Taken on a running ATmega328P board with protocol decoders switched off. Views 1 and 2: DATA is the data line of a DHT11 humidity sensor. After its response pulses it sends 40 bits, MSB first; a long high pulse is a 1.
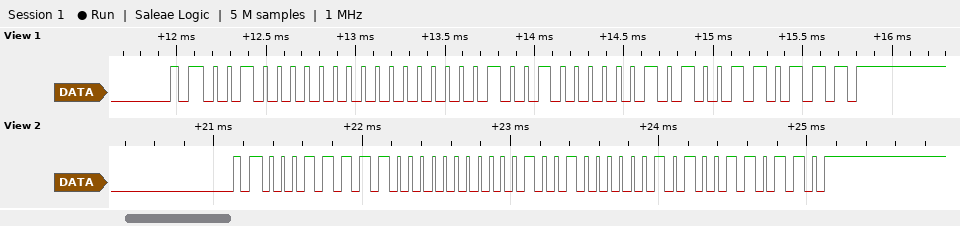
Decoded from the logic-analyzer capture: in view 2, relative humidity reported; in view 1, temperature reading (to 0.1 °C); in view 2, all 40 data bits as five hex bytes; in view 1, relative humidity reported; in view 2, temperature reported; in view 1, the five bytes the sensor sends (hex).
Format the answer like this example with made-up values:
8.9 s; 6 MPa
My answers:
31 %; 18.5 °C; 1F 00 12 05 36; 32 %; 18.5 °C; 20 00 12 05 37
